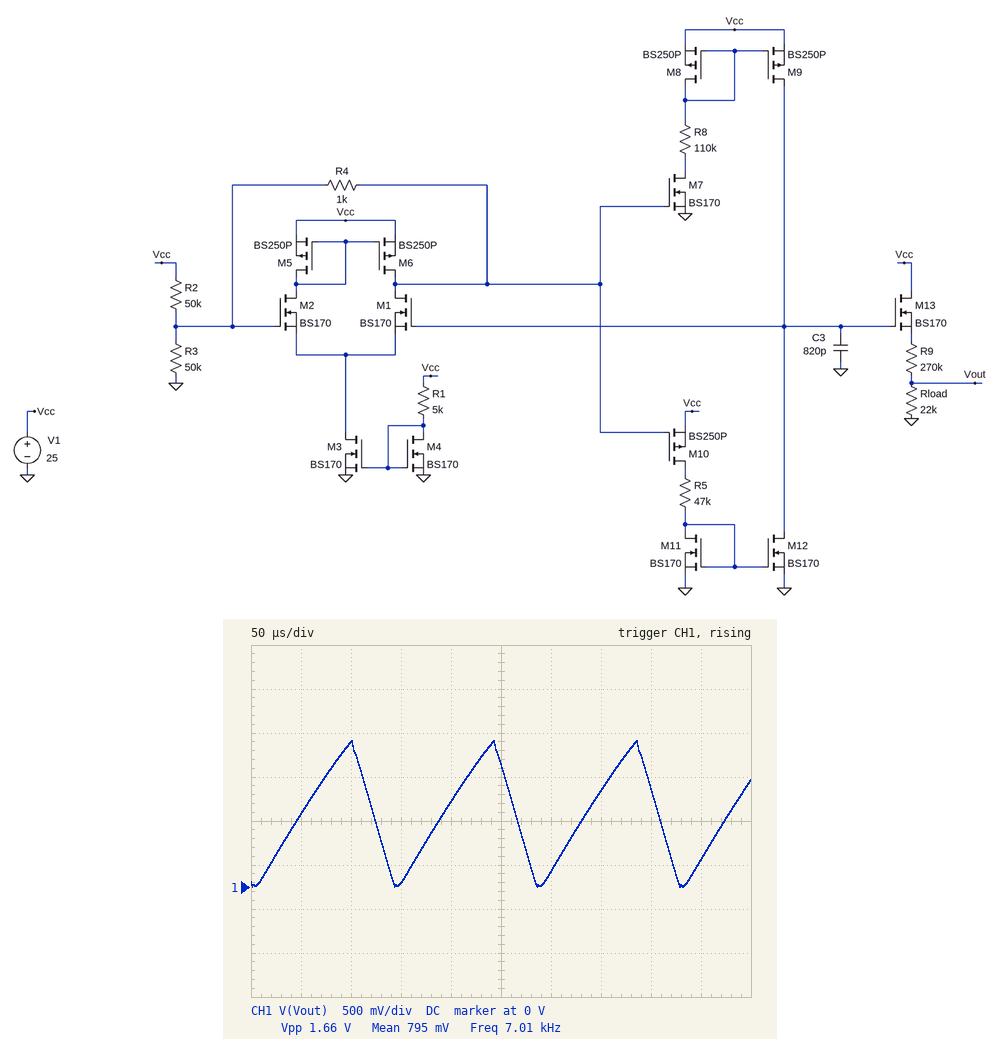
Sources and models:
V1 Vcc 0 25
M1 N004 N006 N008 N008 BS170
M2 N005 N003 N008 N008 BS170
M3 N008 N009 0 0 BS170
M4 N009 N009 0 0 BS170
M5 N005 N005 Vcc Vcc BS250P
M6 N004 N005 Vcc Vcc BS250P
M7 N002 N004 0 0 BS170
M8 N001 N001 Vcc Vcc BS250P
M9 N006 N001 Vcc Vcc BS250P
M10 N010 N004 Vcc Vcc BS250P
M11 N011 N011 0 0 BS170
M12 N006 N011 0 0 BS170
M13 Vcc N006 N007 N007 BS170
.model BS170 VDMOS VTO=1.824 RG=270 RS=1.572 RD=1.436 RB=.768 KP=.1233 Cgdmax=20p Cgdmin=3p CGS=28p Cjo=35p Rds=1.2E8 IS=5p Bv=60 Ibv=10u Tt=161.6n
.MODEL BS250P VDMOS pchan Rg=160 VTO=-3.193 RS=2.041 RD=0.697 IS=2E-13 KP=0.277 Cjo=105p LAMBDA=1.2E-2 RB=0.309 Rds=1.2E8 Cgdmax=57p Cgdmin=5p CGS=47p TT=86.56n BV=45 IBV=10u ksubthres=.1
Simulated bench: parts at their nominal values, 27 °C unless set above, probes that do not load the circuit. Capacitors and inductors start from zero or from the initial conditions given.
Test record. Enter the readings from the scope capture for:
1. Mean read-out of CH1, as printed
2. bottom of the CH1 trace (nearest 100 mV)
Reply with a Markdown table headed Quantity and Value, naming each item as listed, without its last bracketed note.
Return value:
| Quantity | Value |
|---|---|
| Mean read-out of CH1, as printed | 795 mV |
| bottom of the CH1 trace | 0 V |
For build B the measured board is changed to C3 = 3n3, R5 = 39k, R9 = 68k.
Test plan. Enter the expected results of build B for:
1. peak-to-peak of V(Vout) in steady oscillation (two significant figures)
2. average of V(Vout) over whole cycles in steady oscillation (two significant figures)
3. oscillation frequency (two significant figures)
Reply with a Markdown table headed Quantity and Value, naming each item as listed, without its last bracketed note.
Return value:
| Quantity | Value |
|---|---|
| peak-to-peak of V(Vout) in steady oscillation | 5.3 V |
| average of V(Vout) over whole cycles in steady oscillation | 2.7 V |
| oscillation frequency | 2.1 kHz |
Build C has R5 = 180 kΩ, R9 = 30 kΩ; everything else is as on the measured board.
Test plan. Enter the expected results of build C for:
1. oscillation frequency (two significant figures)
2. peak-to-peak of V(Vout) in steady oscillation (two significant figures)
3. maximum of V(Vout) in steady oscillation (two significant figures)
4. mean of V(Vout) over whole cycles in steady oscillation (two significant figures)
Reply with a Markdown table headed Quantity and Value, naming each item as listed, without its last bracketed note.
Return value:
| Quantity | Value |
|---|---|
| oscillation frequency | 3.9 kHz |
| peak-to-peak of V(Vout) in steady oscillation | 9.2 V |
| maximum of V(Vout) in steady oscillation | 9.3 V |
| mean of V(Vout) over whole cycles in steady oscillation | 4.7 V |
